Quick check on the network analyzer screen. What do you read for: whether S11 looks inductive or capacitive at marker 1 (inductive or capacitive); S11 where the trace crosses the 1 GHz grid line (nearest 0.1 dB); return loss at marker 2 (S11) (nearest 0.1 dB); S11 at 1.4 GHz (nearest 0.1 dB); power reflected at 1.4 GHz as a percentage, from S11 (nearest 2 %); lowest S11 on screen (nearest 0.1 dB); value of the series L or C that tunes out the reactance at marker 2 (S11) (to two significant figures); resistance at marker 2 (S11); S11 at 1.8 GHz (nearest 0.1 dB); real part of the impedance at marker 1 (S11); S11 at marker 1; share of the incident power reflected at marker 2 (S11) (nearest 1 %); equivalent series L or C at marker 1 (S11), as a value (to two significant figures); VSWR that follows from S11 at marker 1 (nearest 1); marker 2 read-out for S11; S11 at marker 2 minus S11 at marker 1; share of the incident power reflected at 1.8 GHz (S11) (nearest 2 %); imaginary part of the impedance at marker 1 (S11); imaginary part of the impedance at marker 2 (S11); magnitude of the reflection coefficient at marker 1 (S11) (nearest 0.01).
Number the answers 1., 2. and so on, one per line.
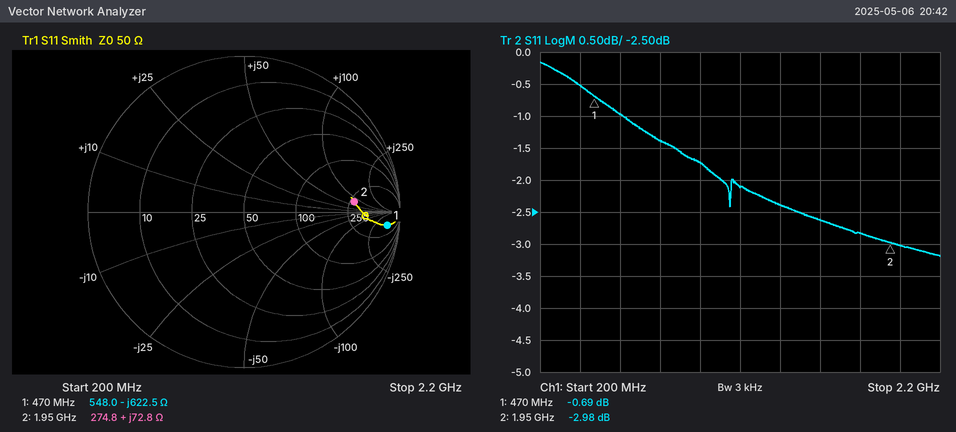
1. capacitive
2. -1.7 dB
3. 3.0 dB
4. -2.4 dB
5. 58 %
6. -3.2 dB
7. 1.1 pF
8. 274.8 Ω
9. -2.8 dB
10. 548.0 Ω
11. -0.69 dB
12. 50 %
13. 540 fF
14. 25
15. -2.98 dB
16. -2.29 dB
17. 52 %
18. -622.5 Ω
19. +72.8 Ω
20. 0.92
